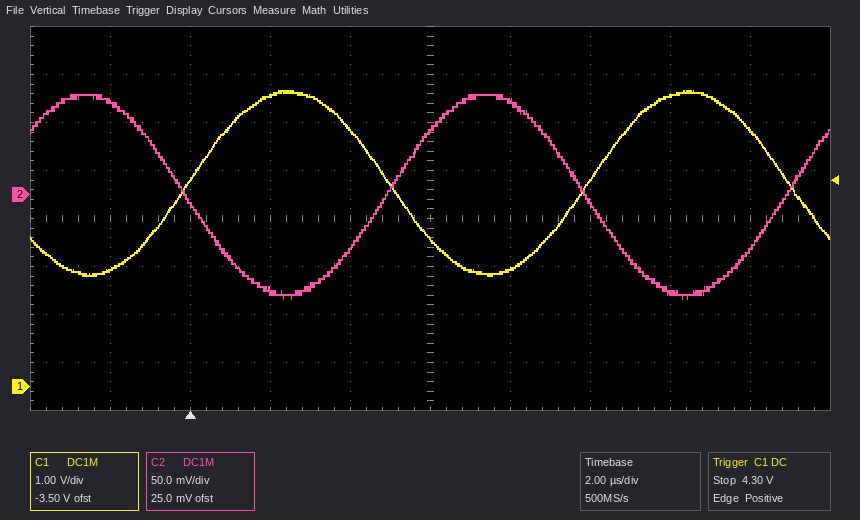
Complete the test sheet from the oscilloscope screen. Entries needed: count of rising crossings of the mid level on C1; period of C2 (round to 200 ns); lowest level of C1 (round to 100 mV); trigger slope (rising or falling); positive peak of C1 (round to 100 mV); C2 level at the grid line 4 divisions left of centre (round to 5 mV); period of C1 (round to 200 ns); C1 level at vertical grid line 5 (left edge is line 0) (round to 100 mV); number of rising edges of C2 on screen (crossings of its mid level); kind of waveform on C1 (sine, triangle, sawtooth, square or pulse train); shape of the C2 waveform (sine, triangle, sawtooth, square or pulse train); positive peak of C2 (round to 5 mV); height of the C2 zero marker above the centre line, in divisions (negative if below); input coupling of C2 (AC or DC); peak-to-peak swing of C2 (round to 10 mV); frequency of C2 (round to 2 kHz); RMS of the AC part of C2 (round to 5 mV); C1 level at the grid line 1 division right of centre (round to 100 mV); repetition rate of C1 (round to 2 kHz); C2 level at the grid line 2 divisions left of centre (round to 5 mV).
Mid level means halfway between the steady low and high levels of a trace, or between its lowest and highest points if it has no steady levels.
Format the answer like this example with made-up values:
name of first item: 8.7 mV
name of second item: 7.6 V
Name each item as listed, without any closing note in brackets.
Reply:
count of rising crossings of the mid level on C1: 2
period of C2: 10.0 µs
lowest level of C1: 2.3 V
trigger slope: rising
positive peak of C1: 6.2 V
C2 level at the grid line 4 divisions left of centre: 95 mV
period of C1: 10.0 µs
C1 level at vertical grid line 5 (left edge is line 0): 3.1 V
number of rising edges of C2 on screen: 2
kind of waveform on C1: sine
shape of the C2 waveform: sine
positive peak of C2: 105 mV
height of the C2 zero marker above the centre line, in divisions: +0.5 div
input coupling of C2: DC
peak-to-peak swing of C2: 210 mV
frequency of C2: 100 kHz
RMS of the AC part of C2: 75 mV
C1 level at the grid line 1 division right of centre: 2.4 V
repetition rate of C1: 100 kHz
C2 level at the grid line 2 divisions left of centre: -100 mV
